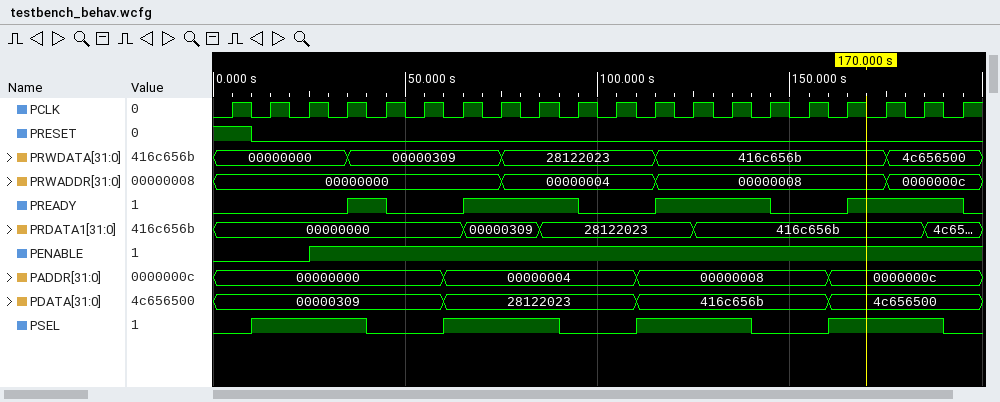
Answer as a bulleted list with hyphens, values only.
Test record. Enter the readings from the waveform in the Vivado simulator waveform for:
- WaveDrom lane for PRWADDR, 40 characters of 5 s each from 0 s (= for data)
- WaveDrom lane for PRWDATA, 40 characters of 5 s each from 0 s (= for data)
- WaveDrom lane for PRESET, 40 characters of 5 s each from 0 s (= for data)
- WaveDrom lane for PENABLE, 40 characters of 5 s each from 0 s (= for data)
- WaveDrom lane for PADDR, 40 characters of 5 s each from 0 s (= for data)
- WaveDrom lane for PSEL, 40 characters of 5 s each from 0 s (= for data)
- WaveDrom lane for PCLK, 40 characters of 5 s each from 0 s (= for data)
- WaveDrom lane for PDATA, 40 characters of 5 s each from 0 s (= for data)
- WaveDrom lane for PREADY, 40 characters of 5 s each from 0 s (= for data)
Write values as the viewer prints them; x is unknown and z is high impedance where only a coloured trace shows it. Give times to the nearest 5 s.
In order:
- {name: 'PRWADDR', wave: '=..............=.......=...........=....', data: '00000000 00000004 00000008 0000000c'}
- {name: 'PRWDATA', wave: '=......=.......=.......=...........=....', data: '00000000 00000309 28122023 416c656b 4c656500'}
- {name: 'PRESET', wave: '1.0.....................................'}
- {name: 'PENABLE', wave: '0....1..................................'}
- {name: 'PADDR', wave: '=...........=.........=.........=.......', data: '00000000 00000004 00000008 0000000c'}
- {name: 'PSEL', wave: '0.1.....0...1.....0...1.....0...1.....0.'}
- {name: 'PCLK', wave: '0101010101010101010101010101010101010101'}
- {name: 'PDATA', wave: '=...........=.........=.........=.......', data: '00000309 28122023 416c656b 4c656500'}
- {name: 'PREADY', wave: '0......1.0...1.....0...1.....0...1.....0'}
